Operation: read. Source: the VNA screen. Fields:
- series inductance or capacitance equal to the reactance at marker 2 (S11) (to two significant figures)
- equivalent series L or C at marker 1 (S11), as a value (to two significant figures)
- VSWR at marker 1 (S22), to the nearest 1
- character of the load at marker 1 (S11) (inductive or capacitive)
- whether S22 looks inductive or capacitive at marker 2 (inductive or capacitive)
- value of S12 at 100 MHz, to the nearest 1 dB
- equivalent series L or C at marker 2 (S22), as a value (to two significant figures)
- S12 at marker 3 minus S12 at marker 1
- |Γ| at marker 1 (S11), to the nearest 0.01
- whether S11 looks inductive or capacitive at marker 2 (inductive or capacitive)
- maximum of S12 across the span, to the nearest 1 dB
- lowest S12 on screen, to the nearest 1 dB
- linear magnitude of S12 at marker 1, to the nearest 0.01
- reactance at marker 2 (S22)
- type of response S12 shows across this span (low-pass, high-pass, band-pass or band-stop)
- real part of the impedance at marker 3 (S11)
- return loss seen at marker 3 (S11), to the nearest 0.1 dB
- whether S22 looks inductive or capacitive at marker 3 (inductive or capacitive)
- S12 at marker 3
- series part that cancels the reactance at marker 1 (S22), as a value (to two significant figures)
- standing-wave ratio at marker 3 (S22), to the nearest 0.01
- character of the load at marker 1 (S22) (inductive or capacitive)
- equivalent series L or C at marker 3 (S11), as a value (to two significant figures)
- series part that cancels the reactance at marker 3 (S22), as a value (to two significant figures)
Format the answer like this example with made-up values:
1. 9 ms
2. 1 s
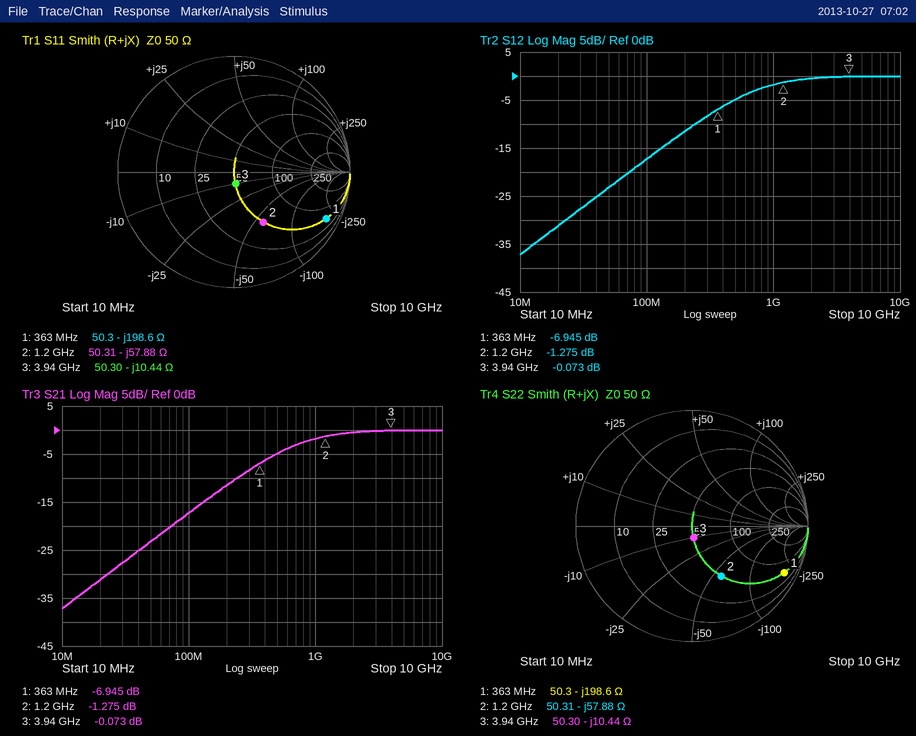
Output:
1. 2.3 pF
2. 2.2 pF
3. 18
4. capacitive
5. capacitive
6. -17 dB
7. 2.3 pF
8. 6.872 dB
9. 0.89
10. capacitive
11. 0 dB
12. -37 dB
13. 0.45
14. -57.88 Ω
15. high-pass
16. 50.30 Ω
17. 19.7 dB
18. capacitive
19. -0.073 dB
20. 87 nH
21. 1.23
22. capacitive
23. 3.9 pF
24. 420 pH
